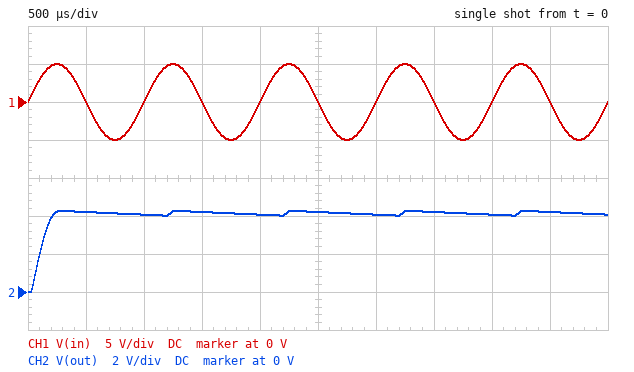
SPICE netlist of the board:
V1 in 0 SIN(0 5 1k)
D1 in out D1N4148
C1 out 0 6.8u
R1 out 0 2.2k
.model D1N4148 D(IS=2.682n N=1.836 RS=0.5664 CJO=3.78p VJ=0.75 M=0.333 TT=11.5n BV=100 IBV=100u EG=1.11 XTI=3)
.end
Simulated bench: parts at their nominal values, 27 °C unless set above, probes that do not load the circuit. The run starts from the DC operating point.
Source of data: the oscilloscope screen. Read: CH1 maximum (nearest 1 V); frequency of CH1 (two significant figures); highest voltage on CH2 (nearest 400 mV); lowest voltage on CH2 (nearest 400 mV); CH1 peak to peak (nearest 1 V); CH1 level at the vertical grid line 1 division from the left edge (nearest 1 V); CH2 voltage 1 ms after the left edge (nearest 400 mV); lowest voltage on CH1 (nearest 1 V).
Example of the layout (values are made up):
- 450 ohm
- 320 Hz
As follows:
- 5 V
- 1.0 kHz
- 4.4 V
- 0 V
- 10 V
- 0 V
- 4.0 V
- -5 V
